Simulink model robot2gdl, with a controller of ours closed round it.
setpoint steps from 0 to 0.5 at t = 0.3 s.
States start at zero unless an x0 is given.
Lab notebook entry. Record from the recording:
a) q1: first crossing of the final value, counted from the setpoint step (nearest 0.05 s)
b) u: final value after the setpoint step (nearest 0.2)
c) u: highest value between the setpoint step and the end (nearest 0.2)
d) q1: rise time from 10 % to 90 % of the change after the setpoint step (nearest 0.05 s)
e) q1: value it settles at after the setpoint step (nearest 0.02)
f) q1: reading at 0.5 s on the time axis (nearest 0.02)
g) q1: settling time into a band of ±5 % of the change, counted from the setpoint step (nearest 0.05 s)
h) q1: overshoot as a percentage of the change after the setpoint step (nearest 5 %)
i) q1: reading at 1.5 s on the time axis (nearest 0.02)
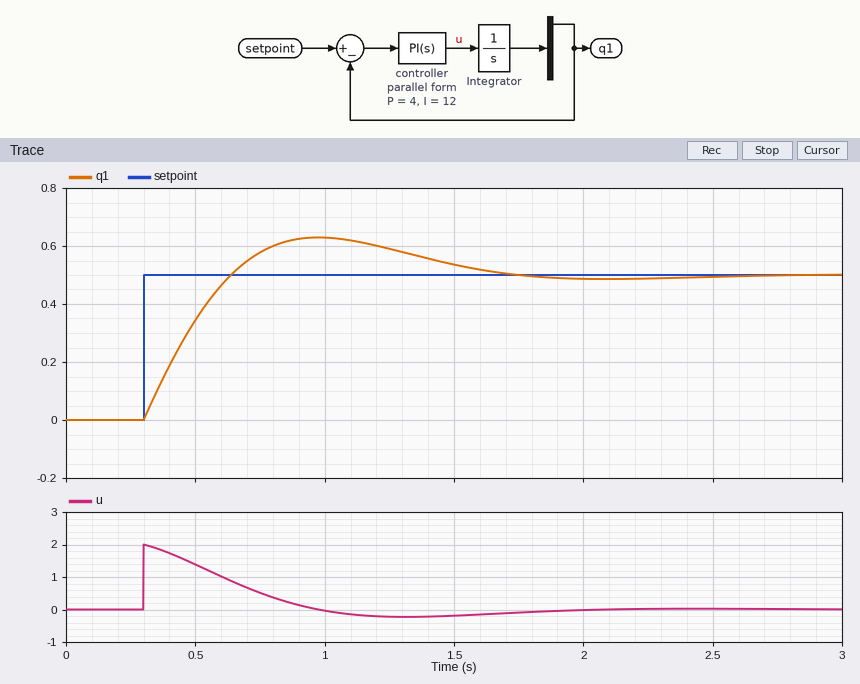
0.35 s
0.0
2.0
0.25 s
0.50
0.34
1.25 s
25 %
0.54
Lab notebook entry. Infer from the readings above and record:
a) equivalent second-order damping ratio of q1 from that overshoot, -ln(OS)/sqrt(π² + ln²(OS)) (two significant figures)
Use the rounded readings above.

0.40
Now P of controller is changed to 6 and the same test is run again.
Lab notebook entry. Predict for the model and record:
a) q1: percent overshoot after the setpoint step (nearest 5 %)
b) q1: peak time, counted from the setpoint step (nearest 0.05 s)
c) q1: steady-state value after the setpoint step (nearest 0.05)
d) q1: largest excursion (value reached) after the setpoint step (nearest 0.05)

15 %
0.60 s
0.50
0.60
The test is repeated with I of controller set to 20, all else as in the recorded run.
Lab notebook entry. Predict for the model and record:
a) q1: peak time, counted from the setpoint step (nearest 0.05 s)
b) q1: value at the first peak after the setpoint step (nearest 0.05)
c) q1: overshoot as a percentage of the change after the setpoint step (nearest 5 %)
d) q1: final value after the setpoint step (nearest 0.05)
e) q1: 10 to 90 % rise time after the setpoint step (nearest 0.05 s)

0.55 s
0.65
35 %
0.50
0.20 s
